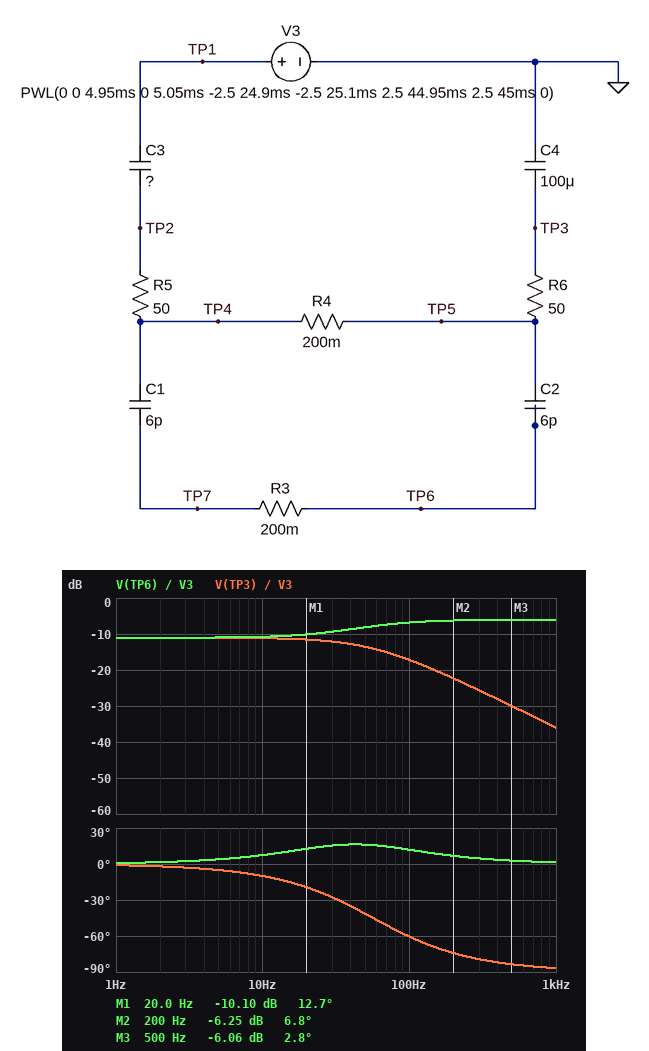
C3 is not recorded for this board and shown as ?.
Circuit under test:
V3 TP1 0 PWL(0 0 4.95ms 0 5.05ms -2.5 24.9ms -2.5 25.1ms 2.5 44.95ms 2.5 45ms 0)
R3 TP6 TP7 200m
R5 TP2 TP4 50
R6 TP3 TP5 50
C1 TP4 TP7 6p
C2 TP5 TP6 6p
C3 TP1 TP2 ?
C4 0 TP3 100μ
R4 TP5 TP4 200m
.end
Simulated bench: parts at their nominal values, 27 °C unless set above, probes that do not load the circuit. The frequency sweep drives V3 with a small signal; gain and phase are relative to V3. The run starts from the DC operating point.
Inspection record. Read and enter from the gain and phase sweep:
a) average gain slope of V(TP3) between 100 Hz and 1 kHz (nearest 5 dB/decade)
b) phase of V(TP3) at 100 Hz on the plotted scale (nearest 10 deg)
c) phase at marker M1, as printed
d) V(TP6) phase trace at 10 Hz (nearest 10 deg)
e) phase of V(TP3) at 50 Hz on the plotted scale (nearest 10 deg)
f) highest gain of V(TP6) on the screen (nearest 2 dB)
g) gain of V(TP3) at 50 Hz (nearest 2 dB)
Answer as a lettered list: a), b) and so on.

a) -20 dB/decade
b) -60 deg
c) 12.7 deg
d) 10 deg
e) -40 deg
f) -6 dB
g) -14 dB
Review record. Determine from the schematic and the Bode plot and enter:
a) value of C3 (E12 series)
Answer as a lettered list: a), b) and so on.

a) 39 µF
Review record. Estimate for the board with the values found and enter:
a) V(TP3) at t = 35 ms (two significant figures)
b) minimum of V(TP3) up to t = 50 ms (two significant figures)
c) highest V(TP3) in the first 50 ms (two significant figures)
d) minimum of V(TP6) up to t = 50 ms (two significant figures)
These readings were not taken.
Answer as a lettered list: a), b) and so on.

a) 660 mV
b) -700 mV
c) 700 mV
d) -1.2 V
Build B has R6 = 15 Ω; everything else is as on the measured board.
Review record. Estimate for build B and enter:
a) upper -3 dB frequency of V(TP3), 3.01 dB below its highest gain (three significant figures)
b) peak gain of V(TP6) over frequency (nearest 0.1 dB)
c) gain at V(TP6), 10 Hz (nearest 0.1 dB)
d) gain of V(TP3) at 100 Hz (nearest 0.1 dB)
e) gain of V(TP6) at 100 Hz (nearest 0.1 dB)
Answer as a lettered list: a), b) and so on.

a) 87.0 Hz
b) -11.0 dB
c) -11.1 dB
d) -14.7 dB
e) -11.9 dB
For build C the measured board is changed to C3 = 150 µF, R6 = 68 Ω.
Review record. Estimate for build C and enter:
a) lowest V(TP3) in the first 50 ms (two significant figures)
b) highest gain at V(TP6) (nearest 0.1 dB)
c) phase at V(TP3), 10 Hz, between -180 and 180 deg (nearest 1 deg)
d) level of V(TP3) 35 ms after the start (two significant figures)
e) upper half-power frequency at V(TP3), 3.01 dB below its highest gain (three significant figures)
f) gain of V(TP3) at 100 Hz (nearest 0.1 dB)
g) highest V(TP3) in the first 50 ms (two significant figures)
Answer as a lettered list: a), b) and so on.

a) -1.4 V
b) -4.4 dB
c) -24 deg
d) 790 mV
e) 22.4 Hz
f) -17.6 dB
g) 1.3 V
